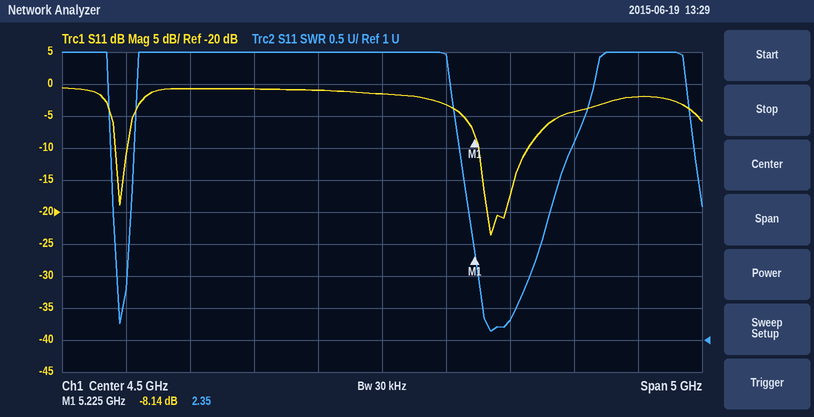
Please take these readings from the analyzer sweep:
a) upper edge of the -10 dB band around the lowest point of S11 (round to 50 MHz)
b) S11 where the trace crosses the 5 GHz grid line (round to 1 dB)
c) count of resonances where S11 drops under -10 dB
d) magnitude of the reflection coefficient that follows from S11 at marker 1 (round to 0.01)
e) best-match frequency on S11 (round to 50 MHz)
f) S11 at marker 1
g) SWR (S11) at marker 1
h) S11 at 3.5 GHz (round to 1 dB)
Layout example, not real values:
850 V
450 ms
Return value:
5.65 GHz
-3 dB
2
0.39
5.35 GHz
-8.14 dB
2.35
-1 dB
